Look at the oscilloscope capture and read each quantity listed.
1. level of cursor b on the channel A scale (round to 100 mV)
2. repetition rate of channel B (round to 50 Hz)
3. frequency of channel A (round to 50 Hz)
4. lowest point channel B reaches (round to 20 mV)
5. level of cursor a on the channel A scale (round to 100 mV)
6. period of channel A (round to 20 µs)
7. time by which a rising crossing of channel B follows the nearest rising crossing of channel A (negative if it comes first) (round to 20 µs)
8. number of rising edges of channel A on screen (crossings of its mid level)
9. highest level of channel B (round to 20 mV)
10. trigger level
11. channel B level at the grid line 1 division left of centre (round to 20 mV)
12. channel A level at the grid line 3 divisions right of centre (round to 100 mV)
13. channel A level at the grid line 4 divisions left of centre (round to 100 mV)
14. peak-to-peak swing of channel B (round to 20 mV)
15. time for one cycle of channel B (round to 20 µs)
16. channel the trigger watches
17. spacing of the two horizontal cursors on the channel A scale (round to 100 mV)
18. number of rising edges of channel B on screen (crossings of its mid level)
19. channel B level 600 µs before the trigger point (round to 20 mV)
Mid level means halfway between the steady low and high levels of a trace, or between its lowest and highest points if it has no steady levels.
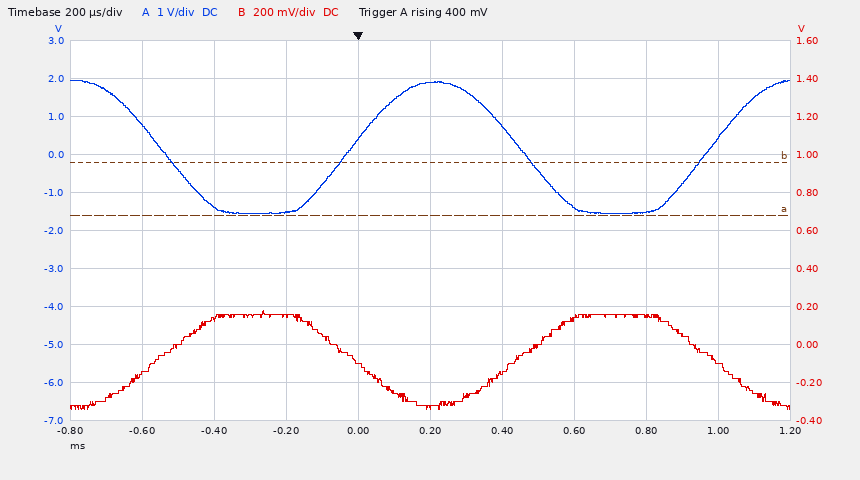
-200 mV
1.00 kHz
1.00 kHz
-340 mV
-1.6 V
1.00 ms
+460 µs
2
180 mV
400 mV
-100 mV
-1.5 V
800 mV
520 mV
1.00 ms
channel A
1.4 V
2
-160 mV
